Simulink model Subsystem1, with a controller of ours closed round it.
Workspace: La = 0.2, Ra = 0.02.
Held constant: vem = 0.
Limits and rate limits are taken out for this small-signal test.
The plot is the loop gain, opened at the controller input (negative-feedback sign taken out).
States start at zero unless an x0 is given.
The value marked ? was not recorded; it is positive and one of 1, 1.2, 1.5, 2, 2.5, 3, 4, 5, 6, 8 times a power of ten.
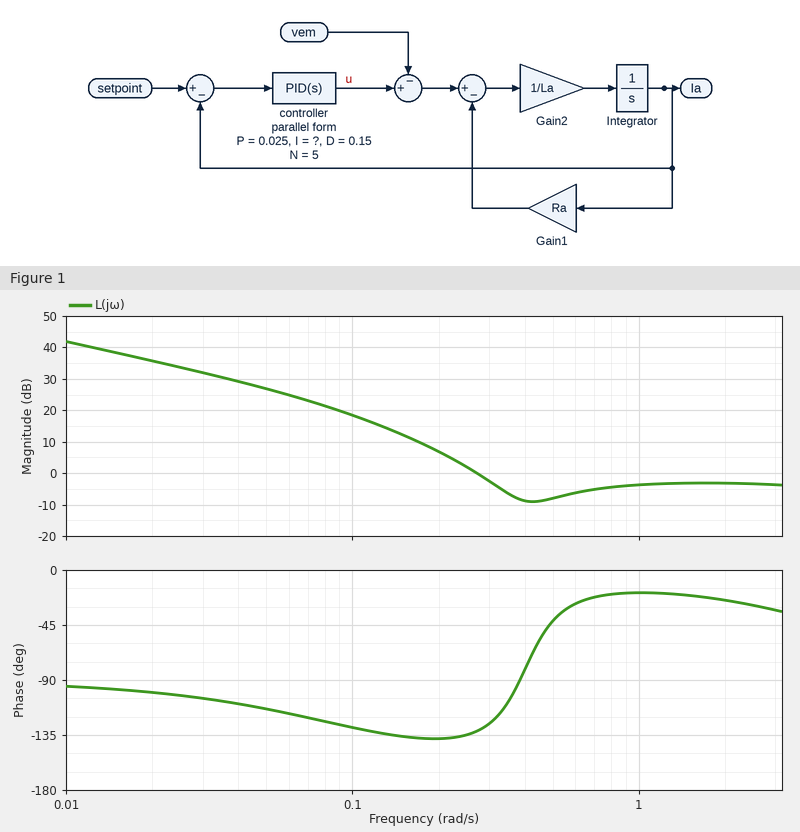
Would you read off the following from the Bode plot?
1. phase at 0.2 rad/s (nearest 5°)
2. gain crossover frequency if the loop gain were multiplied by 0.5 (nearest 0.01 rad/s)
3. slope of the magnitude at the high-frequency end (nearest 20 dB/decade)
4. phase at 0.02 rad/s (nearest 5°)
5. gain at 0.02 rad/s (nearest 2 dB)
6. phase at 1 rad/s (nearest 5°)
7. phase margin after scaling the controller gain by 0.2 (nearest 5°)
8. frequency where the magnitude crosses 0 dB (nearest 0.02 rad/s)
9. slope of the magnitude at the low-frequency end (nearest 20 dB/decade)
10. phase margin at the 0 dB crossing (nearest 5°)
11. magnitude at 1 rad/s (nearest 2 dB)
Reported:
-140°
0.21 rad/s
0 dB/decade
-100°
36 dB
-20°
45°
0.28 rad/s
-20 dB/decade
50°
-4 dB
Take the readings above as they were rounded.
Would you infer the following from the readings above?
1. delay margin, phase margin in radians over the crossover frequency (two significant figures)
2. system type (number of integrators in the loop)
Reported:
3.1 s
1
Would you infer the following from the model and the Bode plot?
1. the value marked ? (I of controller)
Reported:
0.025
